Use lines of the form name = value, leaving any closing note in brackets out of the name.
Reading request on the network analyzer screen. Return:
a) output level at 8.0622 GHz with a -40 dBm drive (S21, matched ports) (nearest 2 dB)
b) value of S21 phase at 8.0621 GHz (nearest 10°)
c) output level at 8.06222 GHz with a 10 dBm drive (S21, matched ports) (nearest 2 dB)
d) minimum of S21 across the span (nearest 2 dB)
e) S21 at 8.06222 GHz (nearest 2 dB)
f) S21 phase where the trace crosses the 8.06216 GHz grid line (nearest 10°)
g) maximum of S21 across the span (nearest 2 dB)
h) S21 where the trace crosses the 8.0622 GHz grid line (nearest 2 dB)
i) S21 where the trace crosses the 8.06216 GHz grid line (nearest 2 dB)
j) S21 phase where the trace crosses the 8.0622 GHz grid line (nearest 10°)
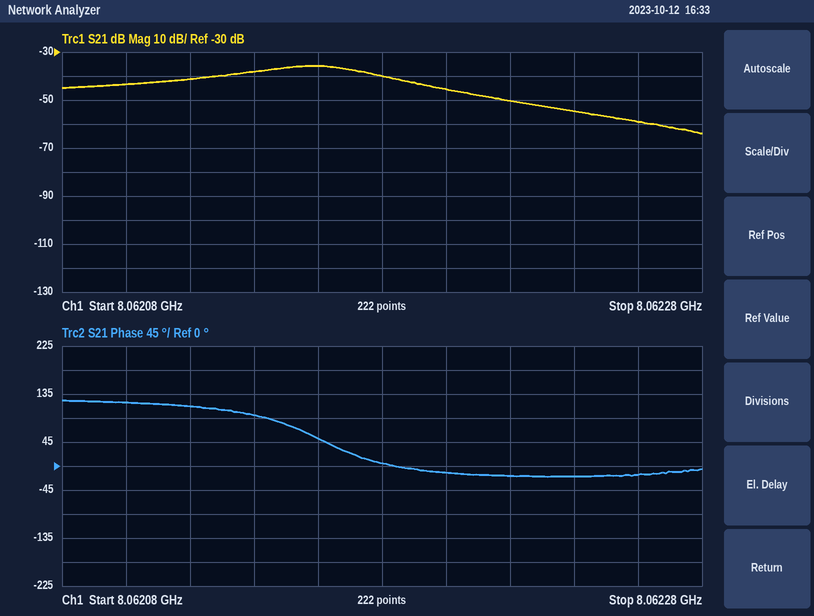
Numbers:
output level at 8.0622 GHz with a -40 dBm drive (S21, matched ports) = -86 dBm
value of S21 phase at 8.0621 GHz = 120°
output level at 8.06222 GHz with a 10 dBm drive (S21, matched ports) = -40 dBm
minimum of S21 across the span = -64 dB
S21 at 8.06222 GHz = -50 dB
S21 phase where the trace crosses the 8.06216 GHz grid line = 50°
maximum of S21 across the span = -36 dB
S21 where the trace crosses the 8.0622 GHz grid line = -46 dB
S21 where the trace crosses the 8.06216 GHz grid line = -36 dB
S21 phase where the trace crosses the 8.0622 GHz grid line = -10°
